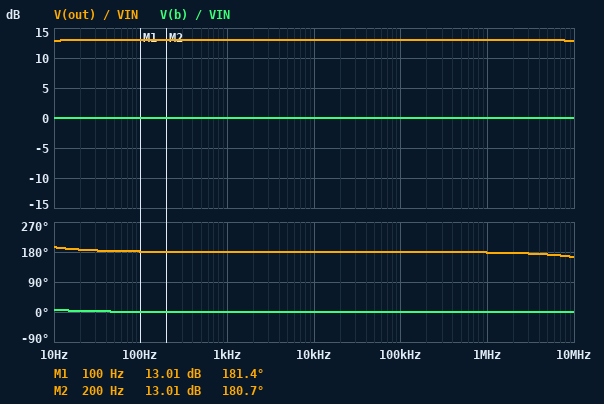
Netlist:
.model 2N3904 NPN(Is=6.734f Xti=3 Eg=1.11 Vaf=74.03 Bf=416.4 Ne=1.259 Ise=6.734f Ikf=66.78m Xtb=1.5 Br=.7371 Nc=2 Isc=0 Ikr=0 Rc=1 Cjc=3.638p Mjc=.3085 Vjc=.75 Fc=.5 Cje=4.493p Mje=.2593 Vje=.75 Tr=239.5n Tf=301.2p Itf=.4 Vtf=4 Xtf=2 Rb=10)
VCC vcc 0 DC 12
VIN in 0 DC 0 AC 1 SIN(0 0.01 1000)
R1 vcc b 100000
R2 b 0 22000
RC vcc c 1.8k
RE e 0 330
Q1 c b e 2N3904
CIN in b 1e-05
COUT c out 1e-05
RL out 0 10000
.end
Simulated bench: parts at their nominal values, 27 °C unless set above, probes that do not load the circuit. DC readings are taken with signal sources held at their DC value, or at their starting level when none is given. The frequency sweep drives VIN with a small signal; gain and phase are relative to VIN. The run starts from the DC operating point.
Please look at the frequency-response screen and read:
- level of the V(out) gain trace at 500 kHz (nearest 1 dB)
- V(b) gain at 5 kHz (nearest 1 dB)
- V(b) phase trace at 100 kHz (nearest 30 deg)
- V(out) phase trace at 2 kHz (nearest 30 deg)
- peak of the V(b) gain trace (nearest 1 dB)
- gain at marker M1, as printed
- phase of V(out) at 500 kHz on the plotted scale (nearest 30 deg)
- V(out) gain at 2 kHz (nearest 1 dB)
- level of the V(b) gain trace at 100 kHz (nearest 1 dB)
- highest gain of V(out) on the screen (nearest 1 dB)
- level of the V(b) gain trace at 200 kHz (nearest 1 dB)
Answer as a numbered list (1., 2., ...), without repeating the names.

1. 13 dB
2. 0 dB
3. 0 deg
4. 180 deg
5. 0 dB
6. 13.01 dB
7. 180 deg
8. 13 dB
9. 0 dB
10. 13 dB
11. 0 dB
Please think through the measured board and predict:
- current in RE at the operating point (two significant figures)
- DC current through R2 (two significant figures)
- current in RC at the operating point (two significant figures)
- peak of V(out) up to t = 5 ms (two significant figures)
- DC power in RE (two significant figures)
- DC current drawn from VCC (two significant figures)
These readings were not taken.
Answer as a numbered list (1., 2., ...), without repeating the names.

1. 3.3 mA
2. 81 µA
3. 3.3 mA
4. 45 mV
5. 3.6 mW
6. 3.4 mA
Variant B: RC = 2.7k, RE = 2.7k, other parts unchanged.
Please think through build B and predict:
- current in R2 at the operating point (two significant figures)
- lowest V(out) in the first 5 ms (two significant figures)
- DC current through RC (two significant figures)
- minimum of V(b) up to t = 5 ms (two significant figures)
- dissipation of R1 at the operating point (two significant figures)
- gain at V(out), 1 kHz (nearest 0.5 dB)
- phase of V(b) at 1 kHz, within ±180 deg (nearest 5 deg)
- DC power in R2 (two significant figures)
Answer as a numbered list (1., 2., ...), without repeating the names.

1. 95 µA
2. -7.7 mV
3. 530 µA
4. 2.1 V
5. 980 µW
6. -2.5 dB
7. 0 deg
8. 200 µW
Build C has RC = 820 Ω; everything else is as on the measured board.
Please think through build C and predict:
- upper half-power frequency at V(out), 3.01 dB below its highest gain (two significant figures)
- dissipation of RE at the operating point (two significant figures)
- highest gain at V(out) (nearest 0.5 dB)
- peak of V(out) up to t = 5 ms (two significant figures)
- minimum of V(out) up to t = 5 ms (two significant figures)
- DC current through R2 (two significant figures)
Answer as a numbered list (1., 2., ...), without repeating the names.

1. 190 MHz
2. 3.7 mW
3. 7.0 dB
4. 22 mV
5. -22 mV
6. 82 µA
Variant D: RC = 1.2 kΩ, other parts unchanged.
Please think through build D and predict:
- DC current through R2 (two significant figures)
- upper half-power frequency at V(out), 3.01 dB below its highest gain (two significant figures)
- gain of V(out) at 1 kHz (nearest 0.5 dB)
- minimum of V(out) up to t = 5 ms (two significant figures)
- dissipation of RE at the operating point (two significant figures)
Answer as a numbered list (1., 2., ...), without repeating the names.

1. 82 µA
2. 95 MHz
3. 10.0 dB
4. -31 mV
5. 3.7 mW
